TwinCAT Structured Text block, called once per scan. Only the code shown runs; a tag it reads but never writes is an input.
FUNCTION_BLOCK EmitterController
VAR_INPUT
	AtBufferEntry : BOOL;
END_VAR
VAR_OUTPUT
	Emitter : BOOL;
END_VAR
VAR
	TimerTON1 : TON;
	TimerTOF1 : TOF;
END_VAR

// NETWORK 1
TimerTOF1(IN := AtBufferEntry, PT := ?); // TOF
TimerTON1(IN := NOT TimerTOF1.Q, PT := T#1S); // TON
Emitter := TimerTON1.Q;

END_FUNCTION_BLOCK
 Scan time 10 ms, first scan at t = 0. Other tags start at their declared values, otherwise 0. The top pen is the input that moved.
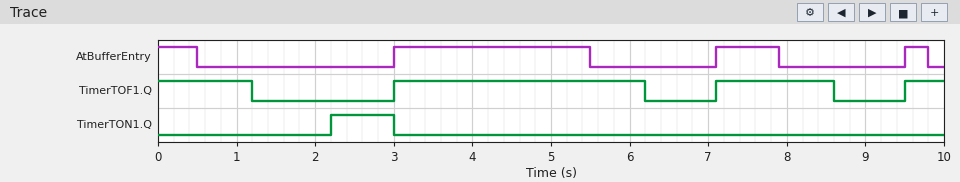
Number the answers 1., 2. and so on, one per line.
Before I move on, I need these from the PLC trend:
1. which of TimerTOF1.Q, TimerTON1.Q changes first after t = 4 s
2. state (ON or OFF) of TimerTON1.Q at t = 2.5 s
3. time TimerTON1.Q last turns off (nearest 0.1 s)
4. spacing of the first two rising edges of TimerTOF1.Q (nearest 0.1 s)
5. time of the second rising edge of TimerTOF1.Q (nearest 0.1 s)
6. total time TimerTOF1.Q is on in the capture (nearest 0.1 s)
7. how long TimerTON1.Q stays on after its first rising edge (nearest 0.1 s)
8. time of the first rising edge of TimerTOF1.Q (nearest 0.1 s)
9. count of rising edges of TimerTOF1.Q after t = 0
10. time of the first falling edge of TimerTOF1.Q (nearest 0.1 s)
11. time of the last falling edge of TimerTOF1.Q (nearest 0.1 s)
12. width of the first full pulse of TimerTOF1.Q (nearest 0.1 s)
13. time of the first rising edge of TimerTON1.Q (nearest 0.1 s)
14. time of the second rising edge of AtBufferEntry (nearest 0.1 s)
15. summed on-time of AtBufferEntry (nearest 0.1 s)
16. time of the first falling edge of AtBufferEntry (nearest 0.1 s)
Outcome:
1. TimerTOF1.Q
2. ON
3. 3.0 s
4. 4.1 s
5. 7.1 s
6. 6.4 s
7. 0.8 s
8. 3.0 s
9. 3
10. 1.2 s
11. 8.6 s
12. 3.2 s
13. 2.2 s
14. 7.1 s
15. 4.1 s
16. 0.5 s
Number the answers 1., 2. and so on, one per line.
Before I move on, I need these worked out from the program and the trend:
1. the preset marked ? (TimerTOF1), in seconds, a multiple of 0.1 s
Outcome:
1. 0.7 s
